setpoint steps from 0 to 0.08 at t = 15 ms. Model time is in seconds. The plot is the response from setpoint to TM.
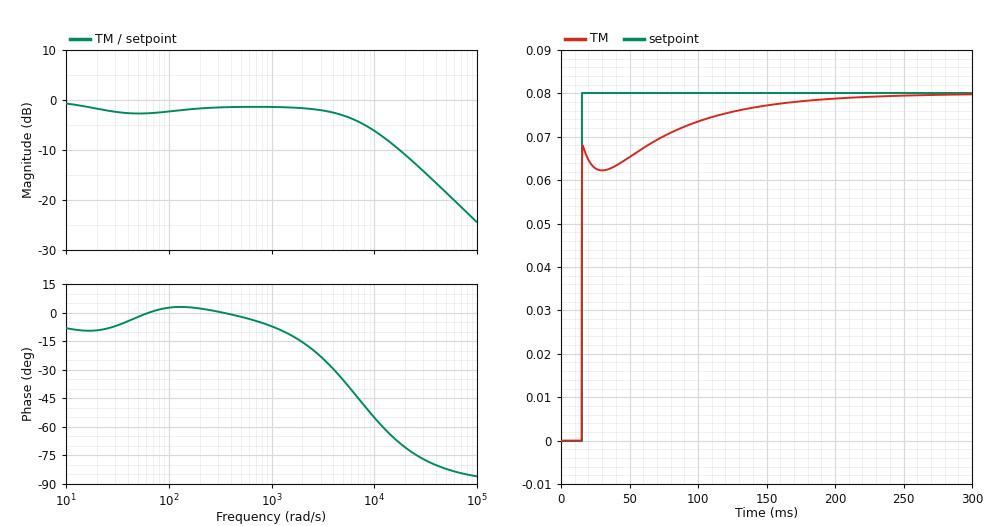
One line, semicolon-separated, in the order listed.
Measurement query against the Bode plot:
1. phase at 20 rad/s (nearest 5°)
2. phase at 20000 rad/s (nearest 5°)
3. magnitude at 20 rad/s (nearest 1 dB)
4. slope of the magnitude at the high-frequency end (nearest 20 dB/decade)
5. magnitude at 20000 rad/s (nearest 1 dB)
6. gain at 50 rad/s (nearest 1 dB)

-10°; -70°; -2 dB; -20 dB/decade; -11 dB; -3 dB
